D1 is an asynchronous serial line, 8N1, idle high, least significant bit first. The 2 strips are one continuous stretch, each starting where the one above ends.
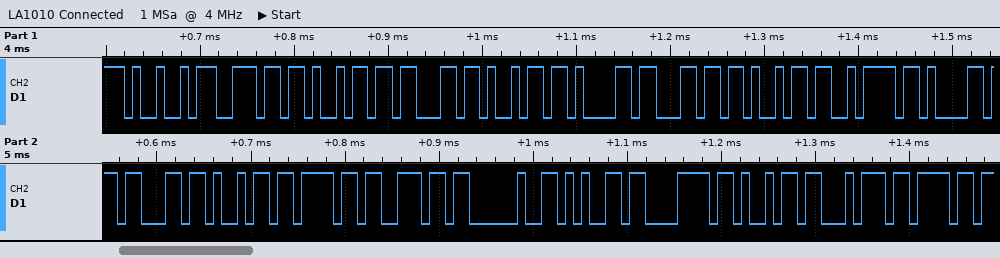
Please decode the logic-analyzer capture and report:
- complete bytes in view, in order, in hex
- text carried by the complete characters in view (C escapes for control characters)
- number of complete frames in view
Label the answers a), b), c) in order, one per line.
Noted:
a) 49 6E 69 63 69 61 6C 69 7A 61 63 69 6F 6E 20 65 78 69 74 6F
b) "Inicializacion exito"
c) 20
